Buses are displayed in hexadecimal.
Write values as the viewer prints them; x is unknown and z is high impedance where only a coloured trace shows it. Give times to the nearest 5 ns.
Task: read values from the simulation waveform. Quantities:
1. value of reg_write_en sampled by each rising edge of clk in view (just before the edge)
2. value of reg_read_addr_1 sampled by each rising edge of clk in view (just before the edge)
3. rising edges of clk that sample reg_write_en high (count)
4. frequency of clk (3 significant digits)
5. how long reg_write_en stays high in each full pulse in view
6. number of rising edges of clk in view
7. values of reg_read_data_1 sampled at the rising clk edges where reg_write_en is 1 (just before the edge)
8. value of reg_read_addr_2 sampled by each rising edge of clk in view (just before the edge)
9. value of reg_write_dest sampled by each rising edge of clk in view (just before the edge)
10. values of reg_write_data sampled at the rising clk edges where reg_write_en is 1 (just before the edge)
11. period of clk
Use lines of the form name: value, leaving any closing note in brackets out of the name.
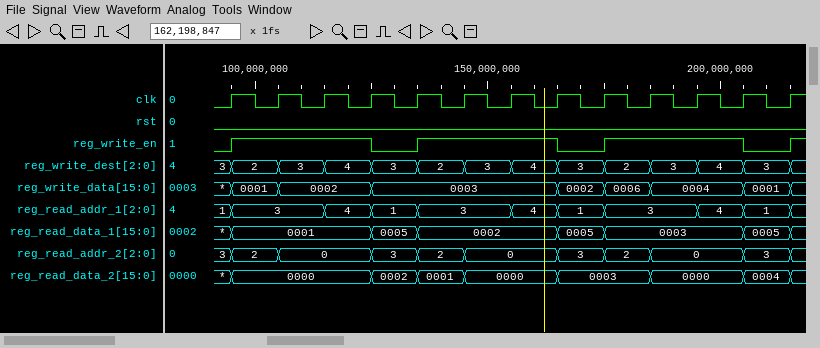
value of reg_write_en sampled by each rising edge of clk in view: 0 1 1 1 0 1 1 1 0 1 1 1 0
value of reg_read_addr_1 sampled by each rising edge of clk in view: 1, 3, 3, 4, 1, 3, 3, 4, 1, 3, 3, 4, 1
rising edges of clk that sample reg_write_en high: 9
frequency of clk: 100 MHz
how long reg_write_en stays high in each full pulse in view: 30 ns, 30 ns, 30 ns
number of rising edges of clk in view: 13
values of reg_read_data_1 sampled at the rising clk edges where reg_write_en is 1: 0001, 0001, 0001, 0002, 0002, 0002, 0003, 0003, 0003
value of reg_read_addr_2 sampled by each rising edge of clk in view: 3, 2, 0, 0, 3, 2, 0, 0, 3, 2, 0, 0, 3
value of reg_write_dest sampled by each rising edge of clk in view: 3, 2, 3, 4, 3, 2, 3, 4, 3, 2, 3, 4, 3
values of reg_write_data sampled at the rising clk edges where reg_write_en is 1: 0001, 0002, 0002, 0003, 0003, 0003, 0006, 0004, 0004
period of clk: 10 ns
